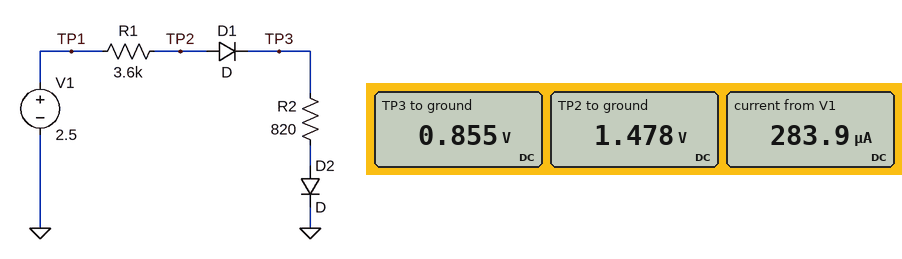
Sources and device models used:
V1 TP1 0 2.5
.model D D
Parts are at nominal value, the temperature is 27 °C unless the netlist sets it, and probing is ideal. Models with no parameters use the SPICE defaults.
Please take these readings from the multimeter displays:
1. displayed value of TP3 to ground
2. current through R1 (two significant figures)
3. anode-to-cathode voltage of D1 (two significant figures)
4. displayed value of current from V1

0.855 V
280 µA
620 mV
283.9 µA
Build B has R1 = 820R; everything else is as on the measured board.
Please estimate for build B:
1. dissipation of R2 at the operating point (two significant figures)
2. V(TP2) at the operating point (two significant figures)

440 µW
1.9 V
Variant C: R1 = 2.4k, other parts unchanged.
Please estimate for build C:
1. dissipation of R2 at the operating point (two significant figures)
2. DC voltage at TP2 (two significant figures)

120 µW
1.6 V
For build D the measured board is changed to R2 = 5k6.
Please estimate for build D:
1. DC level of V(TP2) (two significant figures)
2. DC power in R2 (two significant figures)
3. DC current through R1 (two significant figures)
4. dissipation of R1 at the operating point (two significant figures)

2.0 V
110 µW
140 µA
71 µW
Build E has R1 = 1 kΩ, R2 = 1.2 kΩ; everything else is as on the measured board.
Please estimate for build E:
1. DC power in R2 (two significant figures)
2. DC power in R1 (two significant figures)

370 µW
310 µW
